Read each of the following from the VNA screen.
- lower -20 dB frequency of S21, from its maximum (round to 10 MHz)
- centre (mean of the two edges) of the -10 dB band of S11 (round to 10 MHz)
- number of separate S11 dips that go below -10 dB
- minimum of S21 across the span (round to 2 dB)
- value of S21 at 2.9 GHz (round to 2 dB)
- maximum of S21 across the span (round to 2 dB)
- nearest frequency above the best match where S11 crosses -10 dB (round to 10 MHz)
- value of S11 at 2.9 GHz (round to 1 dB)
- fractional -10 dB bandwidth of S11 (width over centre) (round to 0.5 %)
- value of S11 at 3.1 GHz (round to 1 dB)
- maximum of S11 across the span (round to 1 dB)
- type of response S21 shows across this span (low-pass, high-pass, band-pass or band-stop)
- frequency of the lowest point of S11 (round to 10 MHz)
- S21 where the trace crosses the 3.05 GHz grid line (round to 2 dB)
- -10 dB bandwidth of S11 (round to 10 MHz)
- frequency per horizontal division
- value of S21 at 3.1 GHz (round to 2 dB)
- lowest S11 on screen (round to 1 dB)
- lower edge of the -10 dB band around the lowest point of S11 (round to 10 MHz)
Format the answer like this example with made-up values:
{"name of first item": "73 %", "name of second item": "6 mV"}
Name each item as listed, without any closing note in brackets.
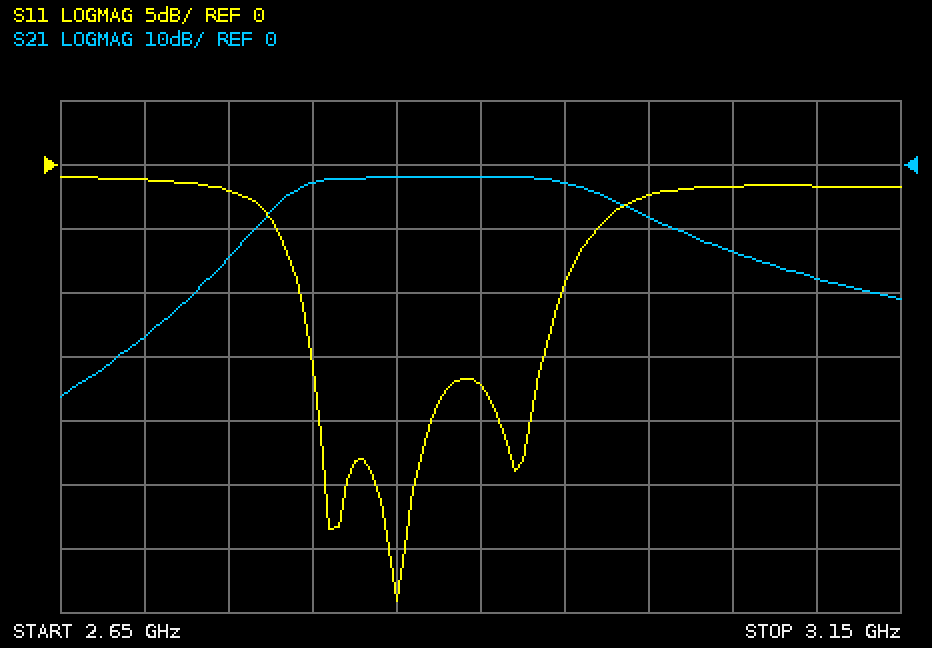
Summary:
{"lower -20 dB frequency of S21, from its maximum": "2.72 GHz", "centre (mean of the two edges) of the -10 dB band of S11": "2.87 GHz", "number of separate S11 dips that go below -10 dB": "3", "minimum of S21 across the span": "-36 dB", "value of S21 at 2.9 GHz": "-2 dB", "maximum of S21 across the span": "-2 dB", "nearest frequency above the best match where S11 crosses -10 dB": "2.95 GHz", "value of S11 at 2.9 GHz": "-17 dB", "fractional -10 dB bandwidth of S11 (width over centre)": "5.5 %", "value of S11 at 3.1 GHz": "-2 dB", "maximum of S11 across the span": "-1 dB", "type of response S21 shows across this span": "band-pass", "frequency of the lowest point of S11": "2.85 GHz", "S21 where the trace crosses the 3.05 GHz grid line": "-14 dB", "-10 dB bandwidth of S11": "160 MHz", "frequency per horizontal division": "50 MHz", "value of S21 at 3.1 GHz": "-18 dB", "lowest S11 on screen": "-34 dB", "lower edge of the -10 dB band around the lowest point of S11": "2.79 GHz"}
